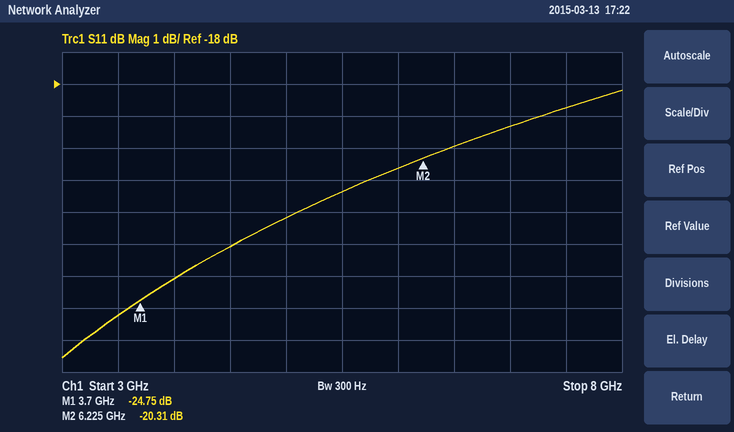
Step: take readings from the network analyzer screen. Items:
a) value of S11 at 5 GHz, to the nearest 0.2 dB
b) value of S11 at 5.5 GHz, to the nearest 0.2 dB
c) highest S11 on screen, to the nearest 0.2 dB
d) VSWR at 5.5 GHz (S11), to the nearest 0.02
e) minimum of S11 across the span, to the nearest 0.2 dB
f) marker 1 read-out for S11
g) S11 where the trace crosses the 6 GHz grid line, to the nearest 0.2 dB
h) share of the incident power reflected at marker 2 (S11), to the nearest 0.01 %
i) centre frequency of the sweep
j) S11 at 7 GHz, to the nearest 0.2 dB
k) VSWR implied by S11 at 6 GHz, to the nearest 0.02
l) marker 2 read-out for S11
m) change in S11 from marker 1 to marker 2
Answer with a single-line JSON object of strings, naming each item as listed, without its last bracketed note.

{"value of S11 at 5 GHz, to the nearest 0.2 dB": "-22.2 dB", "value of S11 at 5.5 GHz, to the nearest 0.2 dB": "-21.4 dB", "highest S11 on screen, to the nearest 0.2 dB": "-18.2 dB", "VSWR at 5.5 GHz (S11), to the nearest 0.02": "1.18", "minimum of S11 across the span, to the nearest 0.2 dB": "-26.6 dB", "marker 1 read-out for S11": "-24.75 dB", "S11 where the trace crosses the 6 GHz grid line, to the nearest 0.2 dB": "-20.6 dB", "share of the incident power reflected at marker 2 (S11), to the nearest 0.01 %": "0.93 %", "centre frequency of the sweep": "5.5 GHz", "S11 at 7 GHz, to the nearest 0.2 dB": "-19.4 dB", "VSWR implied by S11 at 6 GHz, to the nearest 0.02": "1.20", "marker 2 read-out for S11": "-20.31 dB", "change in S11 from marker 1 to marker 2": "4.44 dB"}
